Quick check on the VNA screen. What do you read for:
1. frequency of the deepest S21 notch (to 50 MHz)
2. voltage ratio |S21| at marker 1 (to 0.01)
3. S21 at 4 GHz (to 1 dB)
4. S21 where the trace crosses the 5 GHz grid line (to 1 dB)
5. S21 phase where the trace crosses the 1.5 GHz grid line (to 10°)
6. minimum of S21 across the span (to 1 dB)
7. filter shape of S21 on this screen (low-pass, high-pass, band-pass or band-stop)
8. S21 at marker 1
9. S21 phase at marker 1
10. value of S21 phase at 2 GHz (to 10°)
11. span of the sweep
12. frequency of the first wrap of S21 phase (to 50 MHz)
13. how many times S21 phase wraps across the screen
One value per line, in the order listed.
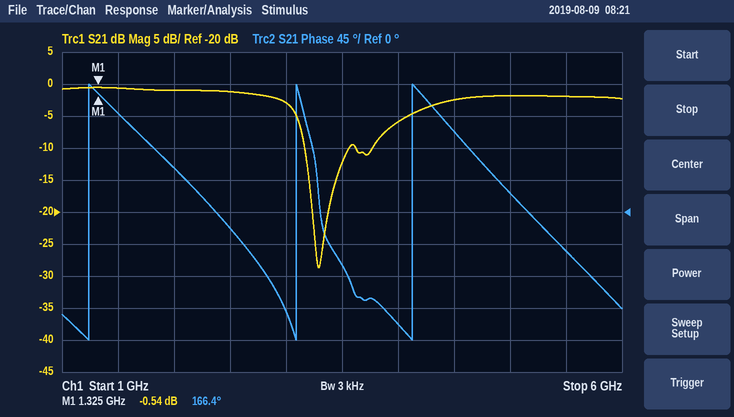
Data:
3.30 GHz
0.94
-6 dB
-2 dB
140°
-29 dB
band-stop
-0.54 dB
166.4°
60°
5 GHz
1.25 GHz
3
